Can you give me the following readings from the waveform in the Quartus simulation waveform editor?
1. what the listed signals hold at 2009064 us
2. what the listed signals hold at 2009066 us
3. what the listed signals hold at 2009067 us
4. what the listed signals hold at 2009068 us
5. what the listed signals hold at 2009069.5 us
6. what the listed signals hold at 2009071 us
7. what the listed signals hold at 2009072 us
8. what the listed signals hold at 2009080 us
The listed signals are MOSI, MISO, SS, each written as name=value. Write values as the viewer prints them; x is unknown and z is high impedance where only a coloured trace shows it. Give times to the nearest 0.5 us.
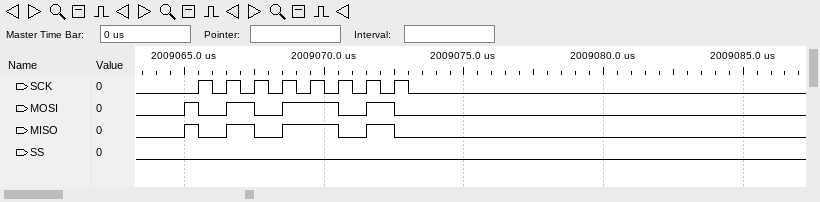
MOSI=0, MISO=0, SS=0
MOSI=0, MISO=0, SS=0
MOSI=1, MISO=1, SS=0
MOSI=0, MISO=0, SS=0
MOSI=1, MISO=1, SS=0
MOSI=0, MISO=0, SS=0
MOSI=1, MISO=1, SS=0
MOSI=0, MISO=0, SS=0
